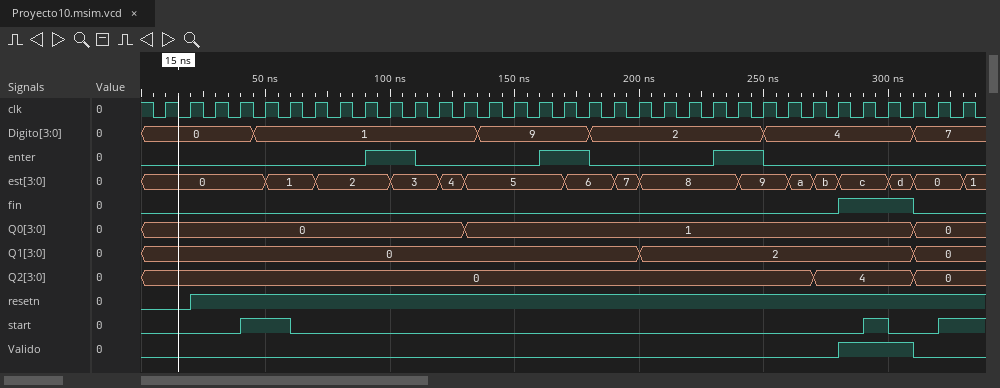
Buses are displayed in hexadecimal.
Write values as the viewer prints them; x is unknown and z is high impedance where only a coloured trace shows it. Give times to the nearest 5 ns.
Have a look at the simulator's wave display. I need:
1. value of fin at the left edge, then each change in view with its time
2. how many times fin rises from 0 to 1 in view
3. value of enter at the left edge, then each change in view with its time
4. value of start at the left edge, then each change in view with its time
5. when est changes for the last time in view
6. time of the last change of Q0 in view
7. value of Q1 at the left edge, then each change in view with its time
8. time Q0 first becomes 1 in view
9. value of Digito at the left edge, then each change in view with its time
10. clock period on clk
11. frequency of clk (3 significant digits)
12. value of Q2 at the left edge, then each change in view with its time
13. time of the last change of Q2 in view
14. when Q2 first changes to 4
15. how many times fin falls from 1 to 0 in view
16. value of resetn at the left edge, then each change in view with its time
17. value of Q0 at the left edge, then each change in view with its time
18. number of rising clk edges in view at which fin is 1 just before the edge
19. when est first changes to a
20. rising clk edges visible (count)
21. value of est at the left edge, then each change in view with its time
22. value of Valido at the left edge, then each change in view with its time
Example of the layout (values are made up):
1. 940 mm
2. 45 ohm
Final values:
1. 0, 1 at 280 ns, 0 at 310 ns
2. 1
3. 0, 1 at 90 ns, 0 at 110 ns, 1 at 160 ns, 0 at 180 ns, 1 at 230 ns, 0 at 250 ns
4. 0, 1 at 40 ns, 0 at 60 ns, 1 at 290 ns, 0 at 300 ns, 1 at 320 ns
5. 330 ns
6. 310 ns
7. 0, 2 at 200 ns, 0 at 310 ns
8. 130 ns
9. 0, 1 at 45 ns, 9 at 135 ns, 2 at 180 ns, 4 at 250 ns, 7 at 310 ns
10. 10 ns
11. 100 MHz
12. 0, 4 at 270 ns, 0 at 310 ns
13. 310 ns
14. 270 ns
15. 1
16. 0, 1 at 20 ns
17. 0, 1 at 130 ns, 0 at 310 ns
18. 3
19. 260 ns
20. 33
21. 0, 1 at 50 ns, 2 at 70 ns, 3 at 100 ns, 4 at 120 ns, 5 at 130 ns, 6 at 170 ns, 7 at 190 ns, 8 at 200 ns, 9 at 240 ns, a at 260 ns, b at 270 ns, c at 280 ns, d at 300 ns, 0 at 310 ns, 1 at 330 ns
22. 0, 1 at 280 ns, 0 at 310 ns
